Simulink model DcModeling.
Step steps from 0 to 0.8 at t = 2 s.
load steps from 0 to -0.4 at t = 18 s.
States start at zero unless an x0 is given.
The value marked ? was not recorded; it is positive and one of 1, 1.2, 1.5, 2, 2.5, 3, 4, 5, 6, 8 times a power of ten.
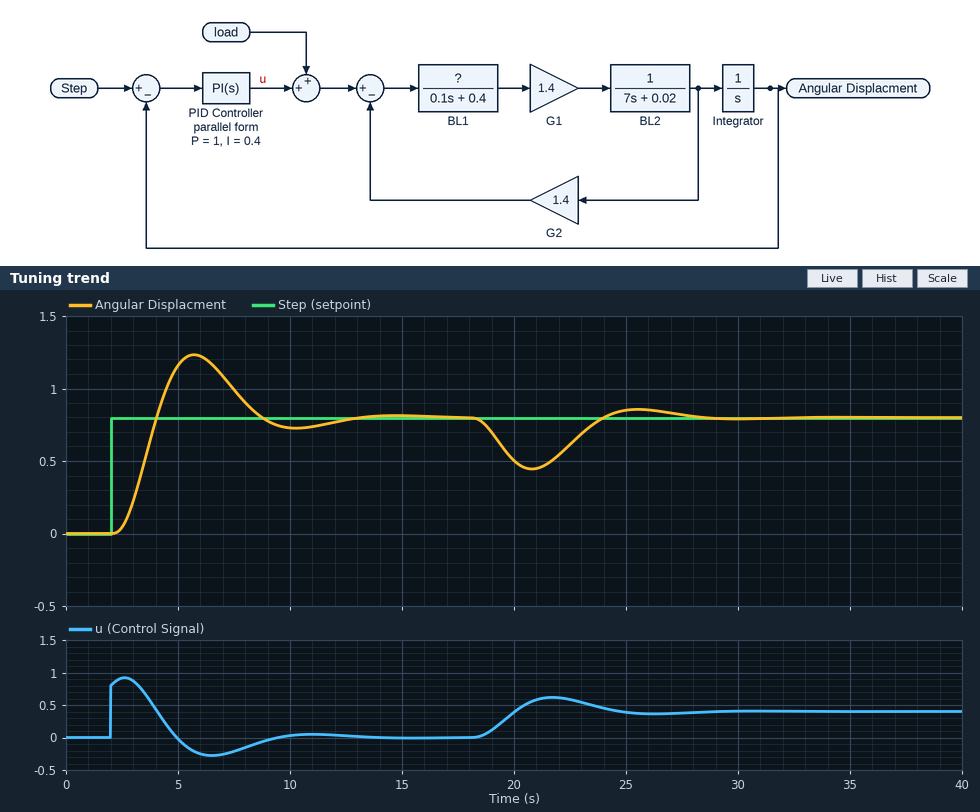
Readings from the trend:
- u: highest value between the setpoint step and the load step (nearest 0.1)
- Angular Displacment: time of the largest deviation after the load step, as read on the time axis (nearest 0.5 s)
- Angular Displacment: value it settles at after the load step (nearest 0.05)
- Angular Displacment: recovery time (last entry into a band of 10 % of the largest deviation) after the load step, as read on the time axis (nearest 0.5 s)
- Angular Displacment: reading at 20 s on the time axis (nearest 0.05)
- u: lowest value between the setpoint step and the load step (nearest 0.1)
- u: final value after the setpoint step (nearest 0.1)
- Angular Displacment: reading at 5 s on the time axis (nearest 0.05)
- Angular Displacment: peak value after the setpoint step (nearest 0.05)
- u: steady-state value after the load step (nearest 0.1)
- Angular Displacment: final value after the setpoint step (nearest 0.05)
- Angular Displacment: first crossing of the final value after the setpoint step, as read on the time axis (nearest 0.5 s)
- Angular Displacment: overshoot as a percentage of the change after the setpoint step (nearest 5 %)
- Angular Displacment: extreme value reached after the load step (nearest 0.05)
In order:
0.9
21.0 s
0.80
27.0 s
0.50
-0.3
0.0
1.15
1.25
0.4
0.80
4.0 s
55 %
0.45
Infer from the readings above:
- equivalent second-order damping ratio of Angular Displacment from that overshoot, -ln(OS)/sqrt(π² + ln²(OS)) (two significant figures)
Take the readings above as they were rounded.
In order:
0.19
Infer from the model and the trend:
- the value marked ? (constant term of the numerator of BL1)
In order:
2
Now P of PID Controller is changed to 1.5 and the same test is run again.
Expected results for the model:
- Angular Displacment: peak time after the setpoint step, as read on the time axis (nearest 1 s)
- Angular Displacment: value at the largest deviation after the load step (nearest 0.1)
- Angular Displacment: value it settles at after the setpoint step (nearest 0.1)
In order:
5 s
0.5
0.8
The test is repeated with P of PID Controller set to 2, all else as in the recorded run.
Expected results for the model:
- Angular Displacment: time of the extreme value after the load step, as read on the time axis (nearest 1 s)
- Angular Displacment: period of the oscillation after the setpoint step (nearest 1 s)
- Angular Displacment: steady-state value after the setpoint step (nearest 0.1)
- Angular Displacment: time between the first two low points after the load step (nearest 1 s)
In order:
20 s
4 s
0.8
4 s
